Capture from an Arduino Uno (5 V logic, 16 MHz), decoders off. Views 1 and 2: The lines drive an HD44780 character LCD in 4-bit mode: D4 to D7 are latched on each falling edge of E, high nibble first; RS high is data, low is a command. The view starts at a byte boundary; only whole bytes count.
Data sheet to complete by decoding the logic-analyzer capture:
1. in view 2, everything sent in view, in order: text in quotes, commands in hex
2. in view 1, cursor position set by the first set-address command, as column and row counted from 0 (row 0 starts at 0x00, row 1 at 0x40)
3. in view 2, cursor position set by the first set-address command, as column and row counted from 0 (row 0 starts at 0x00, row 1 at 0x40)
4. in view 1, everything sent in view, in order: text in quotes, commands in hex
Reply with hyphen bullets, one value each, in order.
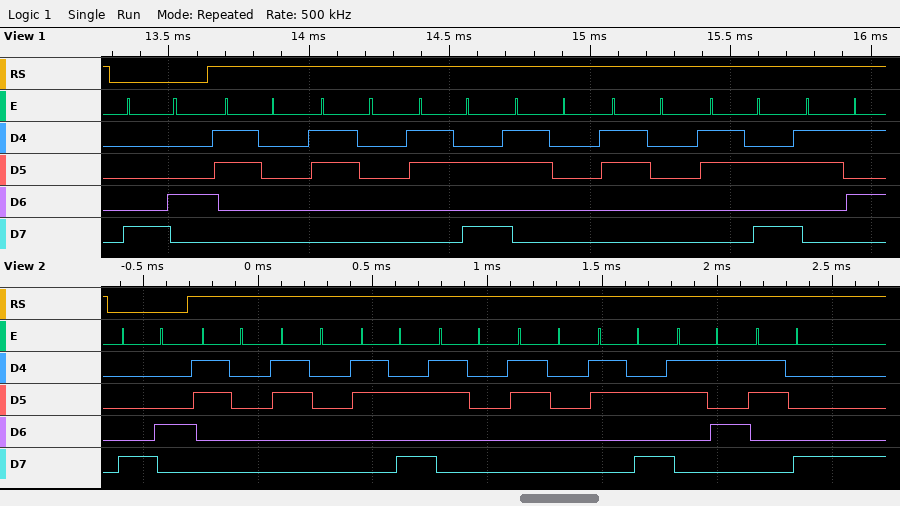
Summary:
- 0x84 "00:00:58"
- column 4, row 0
- column 4, row 0
- 0x84 "00:00:5"
